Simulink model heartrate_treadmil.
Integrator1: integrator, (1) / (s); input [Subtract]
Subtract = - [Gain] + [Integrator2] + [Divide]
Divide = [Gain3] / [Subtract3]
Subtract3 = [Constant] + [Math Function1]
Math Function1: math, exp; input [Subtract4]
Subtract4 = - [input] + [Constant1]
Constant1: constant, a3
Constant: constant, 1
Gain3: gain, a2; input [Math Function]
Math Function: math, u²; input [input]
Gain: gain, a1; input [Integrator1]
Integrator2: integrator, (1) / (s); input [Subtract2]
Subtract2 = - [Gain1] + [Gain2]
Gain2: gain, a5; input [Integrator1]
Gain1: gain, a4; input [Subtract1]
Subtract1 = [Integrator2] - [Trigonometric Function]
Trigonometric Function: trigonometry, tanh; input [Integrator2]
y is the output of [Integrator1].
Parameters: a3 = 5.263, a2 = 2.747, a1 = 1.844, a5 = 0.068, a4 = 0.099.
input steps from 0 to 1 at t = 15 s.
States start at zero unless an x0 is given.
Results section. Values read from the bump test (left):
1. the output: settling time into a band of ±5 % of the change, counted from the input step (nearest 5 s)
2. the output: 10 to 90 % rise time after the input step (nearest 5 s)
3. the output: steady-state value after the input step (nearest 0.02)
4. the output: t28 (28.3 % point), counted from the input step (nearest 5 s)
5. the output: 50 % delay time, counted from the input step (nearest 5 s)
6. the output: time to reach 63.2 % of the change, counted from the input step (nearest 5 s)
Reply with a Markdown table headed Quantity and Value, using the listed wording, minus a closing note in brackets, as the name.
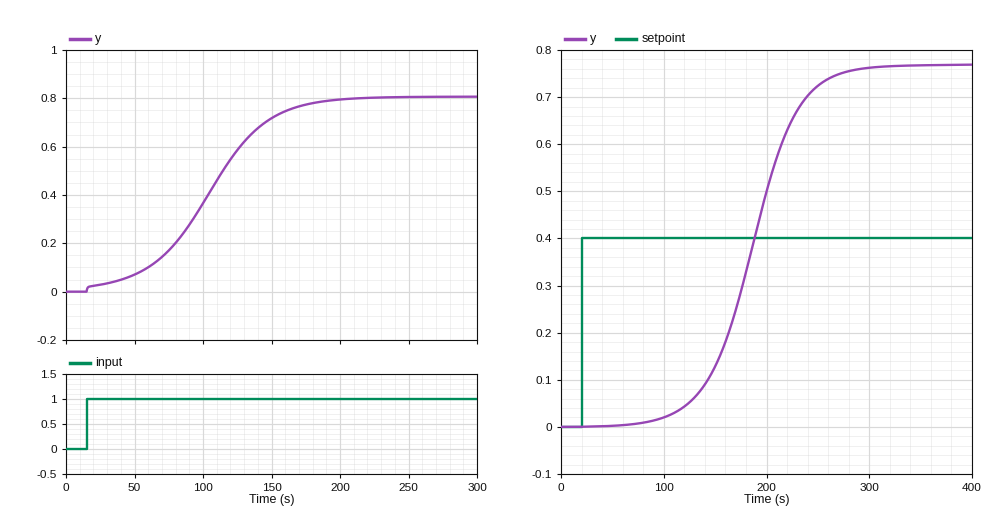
| Quantity | Value |
|---|---|
| the output: settling time into a band of ±5 % of the change, counted from the input step | 155 s |
| the output: 10 to 90 % rise time after the input step | 100 s |
| the output: steady-state value after the input step | 0.80 |
| the output: t28 (28.3 % point), counted from the input step | 70 s |
| the output: 50 % delay time, counted from the input step | 90 s |
| the output: time to reach 63.2 % of the change, counted from the input step | 100 s |
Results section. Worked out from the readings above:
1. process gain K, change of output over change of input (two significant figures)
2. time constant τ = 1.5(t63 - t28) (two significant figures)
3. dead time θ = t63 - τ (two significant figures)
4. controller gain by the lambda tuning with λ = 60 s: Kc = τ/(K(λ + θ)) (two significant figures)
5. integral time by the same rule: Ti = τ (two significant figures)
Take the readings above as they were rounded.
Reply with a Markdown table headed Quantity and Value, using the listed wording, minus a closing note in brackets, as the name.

| Quantity | Value |
|---|---|
| process gain K, change of output over change of input | 0.80 |
| time constant τ = 1.5(t63 - t28) | 45 s |
| dead time θ = t63 - τ | 55 s |
| controller gain by the lambda tuning with λ = 60 s: Kc = τ/(K(λ + θ)) | 0.49 |
| integral time by the same rule: Ti = τ | 45 s |
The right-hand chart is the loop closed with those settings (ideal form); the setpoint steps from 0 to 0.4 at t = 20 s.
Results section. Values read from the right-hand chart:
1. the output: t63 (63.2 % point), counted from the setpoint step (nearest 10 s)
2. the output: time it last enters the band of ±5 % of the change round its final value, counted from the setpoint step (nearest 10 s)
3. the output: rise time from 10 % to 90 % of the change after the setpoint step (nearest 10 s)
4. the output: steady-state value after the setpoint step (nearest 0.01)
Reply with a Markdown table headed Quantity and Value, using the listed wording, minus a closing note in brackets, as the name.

| Quantity | Value |
|---|---|
| the output: t63 (63.2 % point), counted from the setpoint step | 180 s |
| the output: time it last enters the band of ±5 % of the change round its final value, counted from the setpoint step | 230 s |
| the output: rise time from 10 % to 90 % of the change after the setpoint step | 100 s |
| the output: steady-state value after the setpoint step | 0.77 |
